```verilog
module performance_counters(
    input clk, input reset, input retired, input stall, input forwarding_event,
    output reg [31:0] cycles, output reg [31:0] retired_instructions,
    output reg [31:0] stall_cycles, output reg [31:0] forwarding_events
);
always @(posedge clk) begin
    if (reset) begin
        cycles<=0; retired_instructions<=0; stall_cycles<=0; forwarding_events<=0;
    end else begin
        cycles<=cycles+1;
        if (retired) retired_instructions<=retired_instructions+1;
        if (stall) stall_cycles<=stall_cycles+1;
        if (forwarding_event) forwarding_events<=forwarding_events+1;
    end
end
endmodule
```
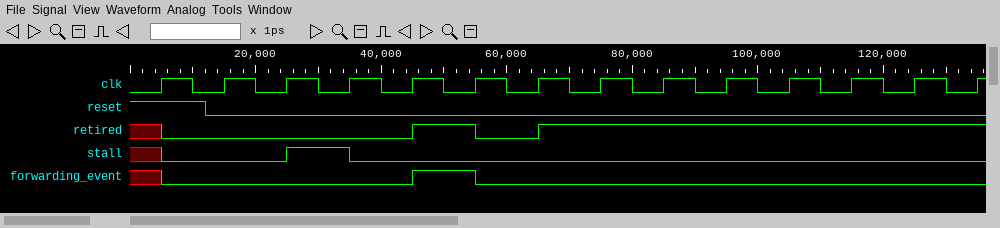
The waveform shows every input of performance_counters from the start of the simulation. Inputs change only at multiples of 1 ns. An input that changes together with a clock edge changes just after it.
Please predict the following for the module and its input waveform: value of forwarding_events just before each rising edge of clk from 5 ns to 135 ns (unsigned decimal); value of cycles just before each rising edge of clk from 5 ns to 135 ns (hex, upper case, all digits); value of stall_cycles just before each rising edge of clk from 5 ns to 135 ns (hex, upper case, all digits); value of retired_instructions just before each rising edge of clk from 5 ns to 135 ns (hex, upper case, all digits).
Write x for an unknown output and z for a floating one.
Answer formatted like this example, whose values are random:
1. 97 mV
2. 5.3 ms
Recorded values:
1. x, 0, 0, 0, 0, 0, 1, 1, 1, 1, 1, 1, 1, 1
2. x, 00000000, 00000001, 00000002, 00000003, 00000004, 00000005, 00000006, 00000007, 00000008, 00000009, 0000000A, 0000000B, 0000000C
3. x, 00000000, 00000000, 00000000, 00000001, 00000001, 00000001, 00000001, 00000001, 00000001, 00000001, 00000001, 00000001, 00000001
4. x, 00000000, 00000000, 00000000, 00000000, 00000000, 00000001, 00000001, 00000002, 00000003, 00000004, 00000005, 00000006, 00000007
